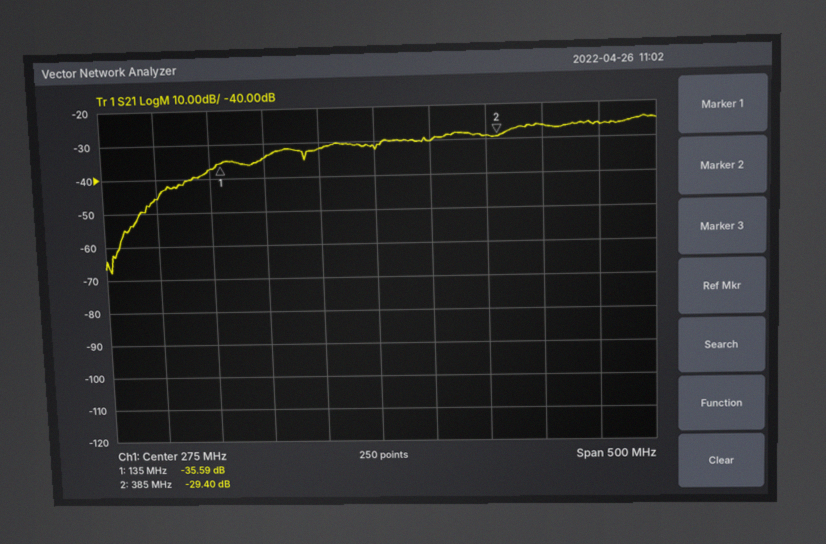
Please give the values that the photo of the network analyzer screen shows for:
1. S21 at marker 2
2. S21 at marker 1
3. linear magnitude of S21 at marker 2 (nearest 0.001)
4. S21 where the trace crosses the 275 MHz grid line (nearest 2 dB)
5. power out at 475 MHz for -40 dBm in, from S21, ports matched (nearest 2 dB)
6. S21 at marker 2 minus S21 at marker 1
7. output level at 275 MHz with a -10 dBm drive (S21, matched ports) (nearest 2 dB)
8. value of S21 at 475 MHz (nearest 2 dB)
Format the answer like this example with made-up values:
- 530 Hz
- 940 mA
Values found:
- -29.40 dB
- -35.59 dB
- 0.034
- -32 dB
- -66 dBm
- 6.19 dB
- -42 dBm
- -26 dB
